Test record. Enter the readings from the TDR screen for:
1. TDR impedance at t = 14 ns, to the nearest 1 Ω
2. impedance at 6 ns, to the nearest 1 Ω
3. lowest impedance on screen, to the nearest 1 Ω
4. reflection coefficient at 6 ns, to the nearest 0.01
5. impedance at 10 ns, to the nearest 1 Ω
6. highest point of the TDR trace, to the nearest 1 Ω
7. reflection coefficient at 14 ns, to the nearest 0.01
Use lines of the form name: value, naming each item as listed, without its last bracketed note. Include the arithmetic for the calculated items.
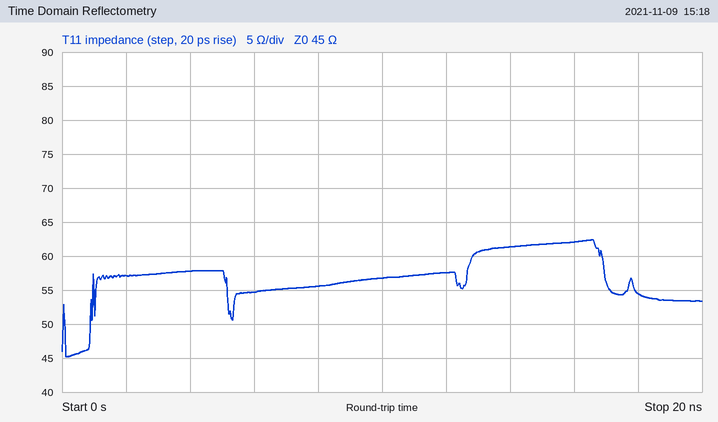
TDR impedance at t = 14 ns, to the nearest 1 Ω: 61 Ω
impedance at 6 ns, to the nearest 1 Ω: 55 Ω
lowest impedance on screen, to the nearest 1 Ω: 45 Ω
reflection coefficient at 6 ns, to the nearest 0.01: (55 − 45)/(55 + 45) ≈ +0.10
impedance at 10 ns, to the nearest 1 Ω: 57 Ω
highest point of the TDR trace, to the nearest 1 Ω: 62 Ω
reflection coefficient at 14 ns, to the nearest 0.01: (61 − 45)/(61 + 45) ≈ +0.15
